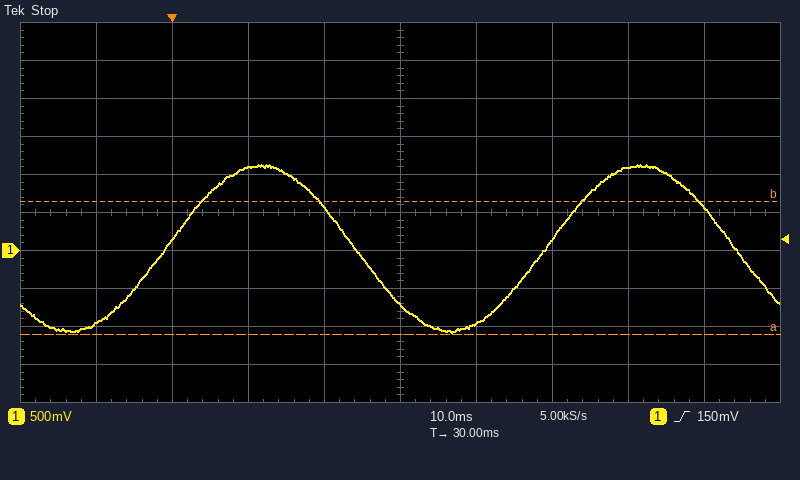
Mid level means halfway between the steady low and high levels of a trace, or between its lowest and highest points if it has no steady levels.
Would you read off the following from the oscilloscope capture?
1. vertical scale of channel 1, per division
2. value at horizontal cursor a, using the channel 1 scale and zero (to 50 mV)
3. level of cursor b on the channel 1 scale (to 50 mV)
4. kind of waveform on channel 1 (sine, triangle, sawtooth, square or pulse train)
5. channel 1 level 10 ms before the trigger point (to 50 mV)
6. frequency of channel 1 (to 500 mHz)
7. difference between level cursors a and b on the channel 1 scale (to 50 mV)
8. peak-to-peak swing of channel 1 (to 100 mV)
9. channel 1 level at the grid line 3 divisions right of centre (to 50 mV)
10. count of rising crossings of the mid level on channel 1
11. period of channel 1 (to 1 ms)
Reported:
500 mV
-1.10 V
650 mV
sine
-950 mV
20.0 Hz
1.75 V
2.20 V
1.10 V
2
50 ms
